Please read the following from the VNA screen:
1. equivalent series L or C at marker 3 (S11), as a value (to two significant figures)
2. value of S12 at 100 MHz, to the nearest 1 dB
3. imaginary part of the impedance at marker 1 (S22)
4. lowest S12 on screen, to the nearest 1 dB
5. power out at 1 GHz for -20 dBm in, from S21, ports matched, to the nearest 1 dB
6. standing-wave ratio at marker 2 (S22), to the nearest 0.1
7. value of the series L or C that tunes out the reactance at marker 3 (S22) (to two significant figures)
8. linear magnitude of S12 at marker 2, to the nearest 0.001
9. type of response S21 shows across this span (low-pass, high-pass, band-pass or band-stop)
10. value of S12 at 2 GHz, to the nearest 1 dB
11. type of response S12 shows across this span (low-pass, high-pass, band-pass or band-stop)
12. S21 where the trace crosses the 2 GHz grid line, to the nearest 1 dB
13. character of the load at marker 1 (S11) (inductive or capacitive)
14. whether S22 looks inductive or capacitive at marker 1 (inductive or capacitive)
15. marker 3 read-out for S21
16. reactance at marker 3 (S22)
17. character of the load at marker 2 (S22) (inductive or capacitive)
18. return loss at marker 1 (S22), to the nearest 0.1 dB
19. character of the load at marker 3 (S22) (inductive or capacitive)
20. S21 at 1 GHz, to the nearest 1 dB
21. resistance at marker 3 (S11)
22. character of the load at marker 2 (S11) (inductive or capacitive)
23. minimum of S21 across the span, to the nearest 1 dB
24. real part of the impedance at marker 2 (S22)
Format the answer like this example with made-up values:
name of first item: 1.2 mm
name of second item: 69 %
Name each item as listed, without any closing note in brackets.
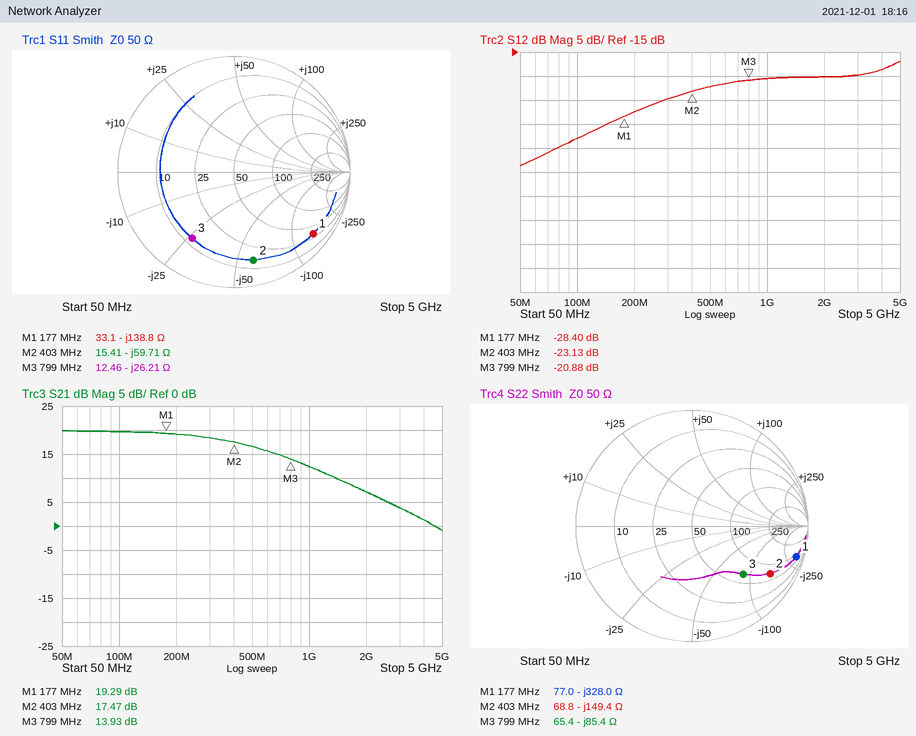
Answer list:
equivalent series L or C at marker 3 (S11), as a value: 7.6 pF
value of S12 at 100 MHz, to the nearest 1 dB: -33 dB
imaginary part of the impedance at marker 1: -328.0 Ω
lowest S12 on screen, to the nearest 1 dB: -39 dB
power out at 1 GHz for -20 dBm in, from S21, ports matched, to the nearest 1 dB: -8 dBm
standing-wave ratio at marker 2 (S22), to the nearest 0.1: 8.5
value of the series L or C that tunes out the reactance at marker 3 (S22): 17 nH
linear magnitude of S12 at marker 2, to the nearest 0.001: 0.070
type of response S21 shows across this span: low-pass
value of S12 at 2 GHz, to the nearest 1 dB: -20 dB
type of response S12 shows across this span: high-pass
S21 where the trace crosses the 2 GHz grid line, to the nearest 1 dB: 7 dB
character of the load at marker 1 (S11): capacitive
whether S22 looks inductive or capacitive at marker 1: capacitive
marker 3 read-out for S21: 13.93 dB
reactance at marker 3: -85.4 Ω
character of the load at marker 2 (S22): capacitive
return loss at marker 1 (S22), to the nearest 0.1 dB: 0.6 dB
character of the load at marker 3 (S22): capacitive
S21 at 1 GHz, to the nearest 1 dB: 12 dB
resistance at marker 3: 12.46 Ω
character of the load at marker 2 (S11): capacitive
minimum of S21 across the span, to the nearest 1 dB: -1 dB
real part of the impedance at marker 2: 68.8 Ω
